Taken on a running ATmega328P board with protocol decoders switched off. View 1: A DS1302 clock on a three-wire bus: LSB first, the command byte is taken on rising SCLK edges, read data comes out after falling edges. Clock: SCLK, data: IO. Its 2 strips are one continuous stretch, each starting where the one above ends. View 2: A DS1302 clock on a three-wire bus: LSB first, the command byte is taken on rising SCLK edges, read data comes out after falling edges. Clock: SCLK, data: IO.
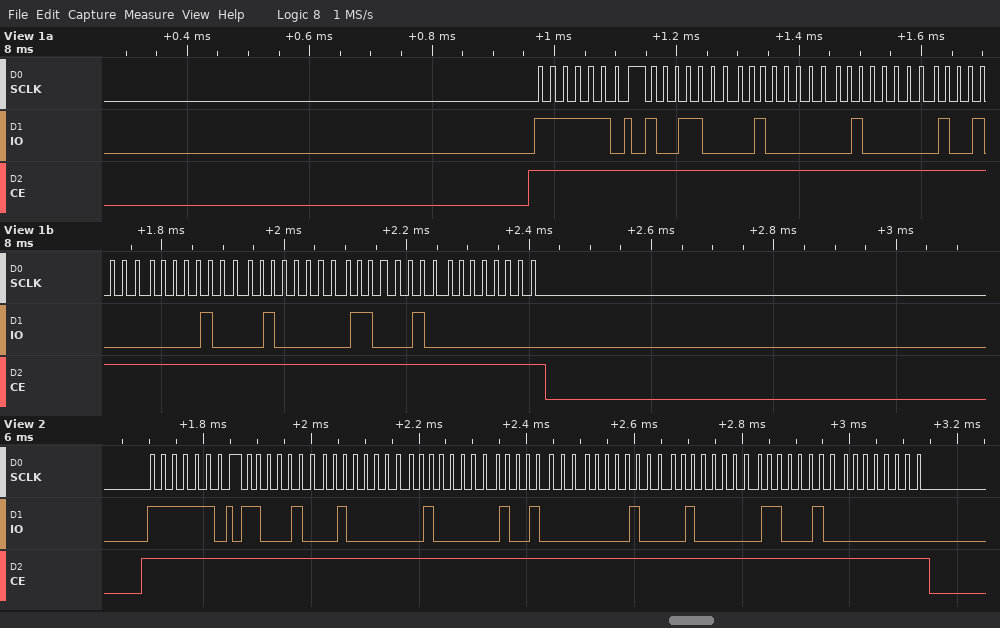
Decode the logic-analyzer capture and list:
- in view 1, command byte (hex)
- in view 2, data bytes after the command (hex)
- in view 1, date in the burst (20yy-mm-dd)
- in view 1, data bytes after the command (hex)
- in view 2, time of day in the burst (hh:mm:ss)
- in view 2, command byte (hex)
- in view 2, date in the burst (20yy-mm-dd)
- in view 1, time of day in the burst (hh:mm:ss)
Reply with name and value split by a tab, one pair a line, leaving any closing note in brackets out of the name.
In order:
in view 1, command byte	0xBF
in view 2, data bytes after the command	23 02 02 09 10 02 23 00
in view 1, date in the burst	2023-10-09
in view 1, data bytes after the command	19 02 02 09 10 02 23 00
in view 2, time of day in the burst	02:02:23
in view 2, command byte	0xBF
in view 2, date in the burst	2023-10-09
in view 1, time of day in the burst	02:02:19
